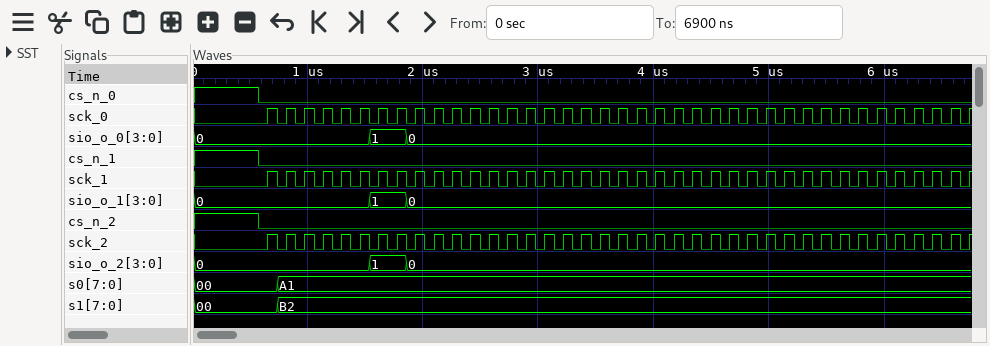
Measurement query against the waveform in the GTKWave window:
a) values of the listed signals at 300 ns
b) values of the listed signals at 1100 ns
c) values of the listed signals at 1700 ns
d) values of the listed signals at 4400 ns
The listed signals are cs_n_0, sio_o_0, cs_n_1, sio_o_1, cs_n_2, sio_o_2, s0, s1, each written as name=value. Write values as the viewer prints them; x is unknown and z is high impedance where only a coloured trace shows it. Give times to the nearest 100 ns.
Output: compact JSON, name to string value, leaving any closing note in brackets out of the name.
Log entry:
{"values of the listed signals at 300 ns": "cs_n_0=1, sio_o_0=0, cs_n_1=1, sio_o_1=0, cs_n_2=1, sio_o_2=0, s0=00, s1=00", "values of the listed signals at 1100 ns": "cs_n_0=0, sio_o_0=0, cs_n_1=0, sio_o_1=0, cs_n_2=0, sio_o_2=0, s0=A1, s1=B2", "values of the listed signals at 1700 ns": "cs_n_0=0, sio_o_0=1, cs_n_1=0, sio_o_1=1, cs_n_2=0, sio_o_2=1, s0=A1, s1=B2", "values of the listed signals at 4400 ns": "cs_n_0=0, sio_o_0=0, cs_n_1=0, sio_o_1=0, cs_n_2=0, sio_o_2=0, s0=A1, s1=B2"}
